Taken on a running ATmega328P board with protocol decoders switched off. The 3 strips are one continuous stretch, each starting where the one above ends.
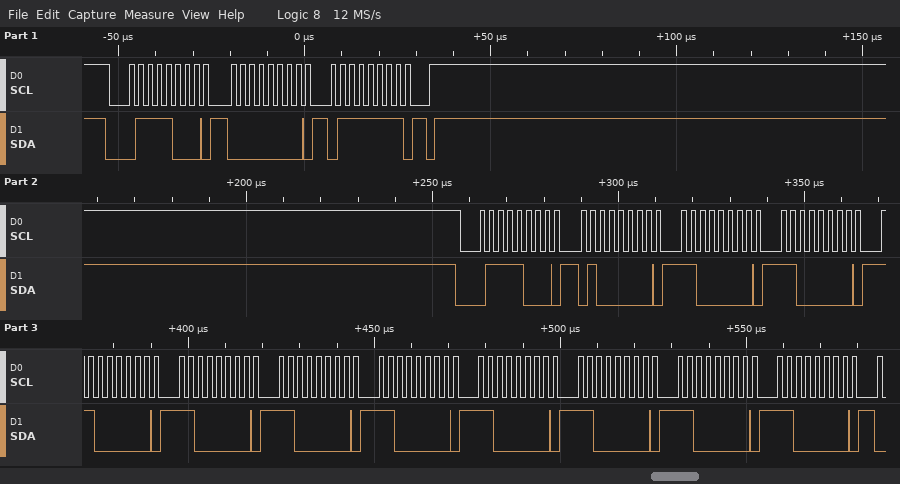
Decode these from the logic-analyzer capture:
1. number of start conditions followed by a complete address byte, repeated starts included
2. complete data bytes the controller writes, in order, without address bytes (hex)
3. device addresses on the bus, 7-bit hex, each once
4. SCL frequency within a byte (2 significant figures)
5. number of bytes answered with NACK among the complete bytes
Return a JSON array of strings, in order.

["2", "00 7F 40 C0 C0 C0 C0 C0 C0 C0 C0 C0 C0", "0x3C", "400 kHz", "0"]
